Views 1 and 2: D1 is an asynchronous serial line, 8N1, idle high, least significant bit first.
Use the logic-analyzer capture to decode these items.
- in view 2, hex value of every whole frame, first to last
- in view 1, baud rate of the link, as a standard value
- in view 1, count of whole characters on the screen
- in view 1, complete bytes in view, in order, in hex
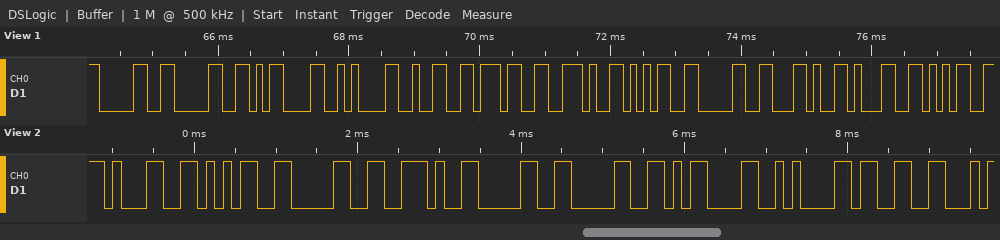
0x31 0x35 0x30 0x2E 0x30 0x30 0x0D 0x0A 0x33
9600 baud
12
0x30 0x30 0x0D 0x0A 0x32 0x37 0x2E 0x35 0x30 0x2C 0x31 0x35
